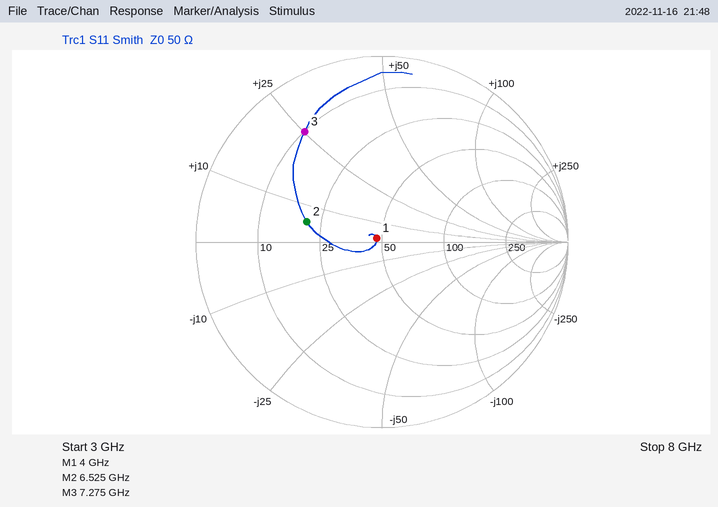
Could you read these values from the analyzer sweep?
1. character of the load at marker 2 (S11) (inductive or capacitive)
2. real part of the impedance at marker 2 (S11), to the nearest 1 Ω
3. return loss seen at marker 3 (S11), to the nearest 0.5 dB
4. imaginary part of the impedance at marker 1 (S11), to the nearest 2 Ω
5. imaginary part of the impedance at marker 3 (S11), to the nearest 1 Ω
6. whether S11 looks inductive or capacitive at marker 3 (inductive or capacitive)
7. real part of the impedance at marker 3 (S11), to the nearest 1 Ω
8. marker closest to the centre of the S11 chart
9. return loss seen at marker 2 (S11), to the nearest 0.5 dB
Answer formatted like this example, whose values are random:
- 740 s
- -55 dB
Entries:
- inductive
- 21 Ω
- 3.0 dB
- +2 Ω
- +25 Ω
- inductive
- 10 Ω
- marker 1
- 7.5 dB
